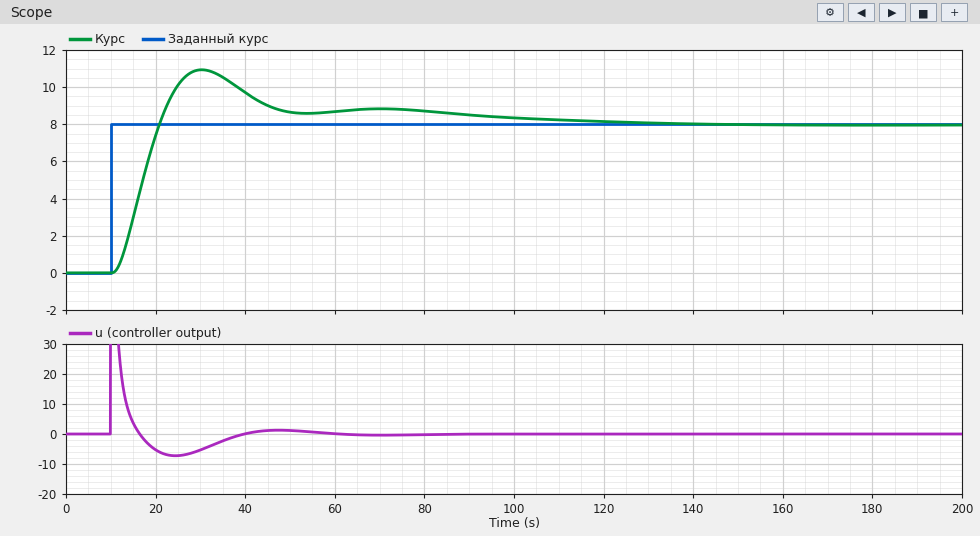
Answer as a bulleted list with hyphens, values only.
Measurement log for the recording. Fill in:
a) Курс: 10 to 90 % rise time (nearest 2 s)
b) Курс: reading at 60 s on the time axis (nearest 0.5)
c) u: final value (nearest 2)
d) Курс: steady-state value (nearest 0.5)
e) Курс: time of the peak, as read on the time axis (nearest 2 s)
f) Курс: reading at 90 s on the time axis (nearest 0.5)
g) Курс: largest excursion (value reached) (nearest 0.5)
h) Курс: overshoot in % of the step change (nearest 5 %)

- 8 s
- 8.5
- 0
- 8.0
- 30 s
- 8.5
- 11.0
- 35 %
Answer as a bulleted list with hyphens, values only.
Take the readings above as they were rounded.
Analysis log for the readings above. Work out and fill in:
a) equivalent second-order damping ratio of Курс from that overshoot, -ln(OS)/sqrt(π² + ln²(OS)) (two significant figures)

- 0.32
